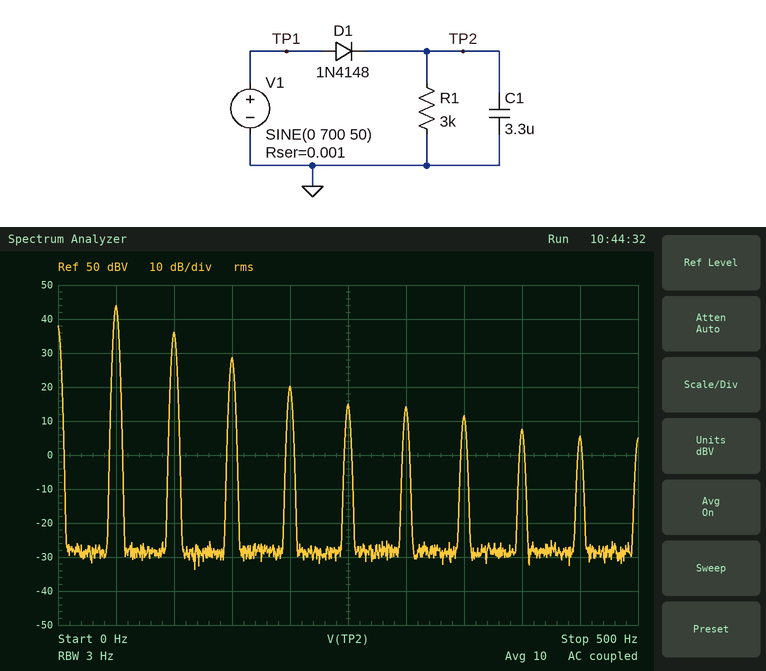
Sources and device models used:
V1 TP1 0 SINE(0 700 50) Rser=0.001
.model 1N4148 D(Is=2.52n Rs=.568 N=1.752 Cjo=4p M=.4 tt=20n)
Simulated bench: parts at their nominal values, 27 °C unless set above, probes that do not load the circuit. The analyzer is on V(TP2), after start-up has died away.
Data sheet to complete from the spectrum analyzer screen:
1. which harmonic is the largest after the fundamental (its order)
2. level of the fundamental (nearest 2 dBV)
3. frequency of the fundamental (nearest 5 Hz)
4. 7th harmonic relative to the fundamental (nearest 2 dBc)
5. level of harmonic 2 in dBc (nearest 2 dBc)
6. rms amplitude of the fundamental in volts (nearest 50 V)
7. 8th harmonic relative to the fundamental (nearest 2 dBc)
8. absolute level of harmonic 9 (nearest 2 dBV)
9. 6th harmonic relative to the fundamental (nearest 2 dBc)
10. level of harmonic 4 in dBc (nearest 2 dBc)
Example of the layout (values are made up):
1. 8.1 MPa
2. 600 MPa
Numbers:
1. 2
2. 44 dBV
3. 50 Hz
4. -32 dBc
5. -8 dBc
6. 150 V
7. -36 dBc
8. 6 dBV
9. -30 dBc
10. -24 dBc
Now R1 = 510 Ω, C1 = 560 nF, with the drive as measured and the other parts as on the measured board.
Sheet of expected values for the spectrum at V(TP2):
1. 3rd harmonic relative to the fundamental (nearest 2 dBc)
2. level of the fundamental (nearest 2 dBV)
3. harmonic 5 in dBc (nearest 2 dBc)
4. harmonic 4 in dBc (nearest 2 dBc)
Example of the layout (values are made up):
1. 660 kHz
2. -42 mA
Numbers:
1. -52 dBc
2. 48 dBV
3. -52 dBc
4. -22 dBc
